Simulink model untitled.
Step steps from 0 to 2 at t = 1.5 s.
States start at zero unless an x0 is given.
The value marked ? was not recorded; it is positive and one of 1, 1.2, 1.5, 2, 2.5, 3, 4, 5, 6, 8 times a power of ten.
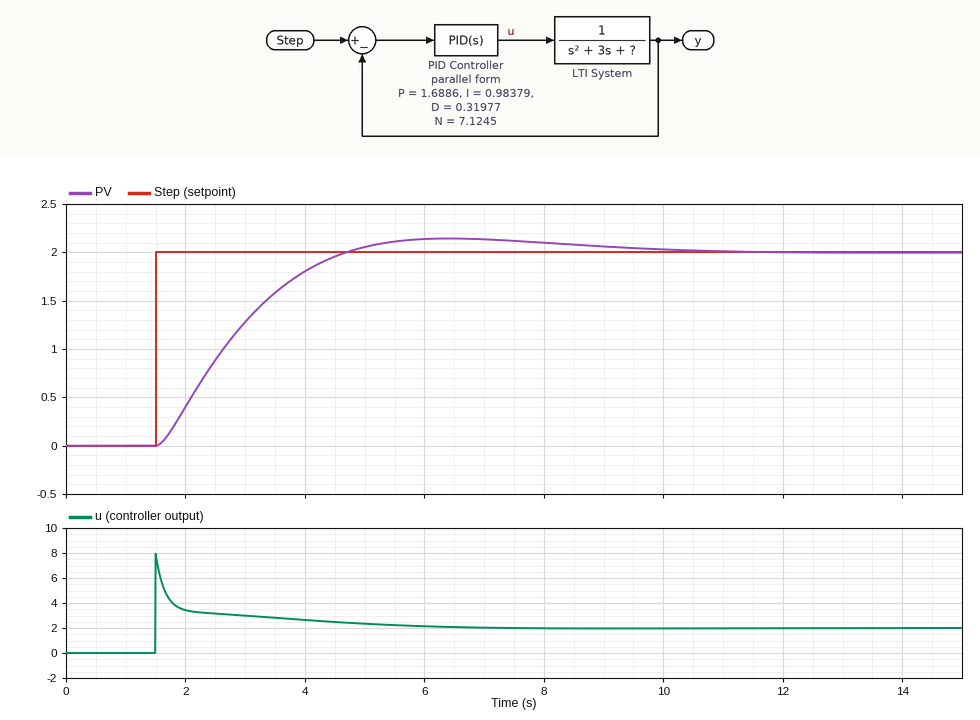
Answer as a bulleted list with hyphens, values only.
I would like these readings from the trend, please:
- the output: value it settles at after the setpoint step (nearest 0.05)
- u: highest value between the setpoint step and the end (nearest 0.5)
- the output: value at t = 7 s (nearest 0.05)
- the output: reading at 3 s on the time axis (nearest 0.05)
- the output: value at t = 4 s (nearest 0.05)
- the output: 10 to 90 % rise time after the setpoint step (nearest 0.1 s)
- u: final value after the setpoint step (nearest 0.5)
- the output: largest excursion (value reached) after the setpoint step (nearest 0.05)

- 2.00
- 8.0
- 2.15
- 1.30
- 1.80
- 2.2 s
- 2.0
- 2.15
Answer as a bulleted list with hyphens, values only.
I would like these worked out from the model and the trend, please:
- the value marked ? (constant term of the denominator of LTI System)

- 1
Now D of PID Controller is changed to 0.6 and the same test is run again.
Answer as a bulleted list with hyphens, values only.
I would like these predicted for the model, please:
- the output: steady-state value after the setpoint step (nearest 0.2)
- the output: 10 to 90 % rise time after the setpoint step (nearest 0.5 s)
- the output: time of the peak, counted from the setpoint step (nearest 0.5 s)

- 2.0
- 2.5 s
- 5.5 s
